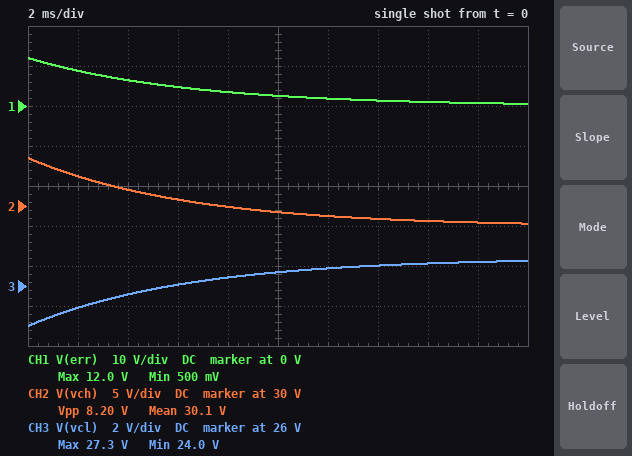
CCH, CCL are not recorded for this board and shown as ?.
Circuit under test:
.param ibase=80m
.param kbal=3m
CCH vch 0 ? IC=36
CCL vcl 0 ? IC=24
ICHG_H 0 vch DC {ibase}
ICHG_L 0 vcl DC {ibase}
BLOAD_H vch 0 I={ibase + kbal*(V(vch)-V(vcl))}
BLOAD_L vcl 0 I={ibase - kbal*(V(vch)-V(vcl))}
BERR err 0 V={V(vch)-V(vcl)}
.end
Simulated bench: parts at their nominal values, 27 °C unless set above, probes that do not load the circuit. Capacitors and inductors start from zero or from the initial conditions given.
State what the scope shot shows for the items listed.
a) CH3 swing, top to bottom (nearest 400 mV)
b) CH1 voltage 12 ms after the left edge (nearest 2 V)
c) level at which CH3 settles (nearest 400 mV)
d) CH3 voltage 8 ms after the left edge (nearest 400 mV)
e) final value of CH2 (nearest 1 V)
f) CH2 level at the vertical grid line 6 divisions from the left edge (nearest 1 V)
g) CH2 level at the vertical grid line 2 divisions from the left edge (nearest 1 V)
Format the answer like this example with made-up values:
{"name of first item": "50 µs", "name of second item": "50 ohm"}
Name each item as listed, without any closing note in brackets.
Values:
{"CH3 swing, top to bottom": "3.2 V", "CH1 voltage 12 ms after the left edge": "2 V", "level at which CH3 settles": "27.2 V", "CH3 voltage 8 ms after the left edge": "26.4 V", "final value of CH2": "28 V", "CH2 level at the vertical grid line 6 divisions from the left edge": "29 V", "CH2 level at the vertical grid line 2 divisions from the left edge": "32 V"}
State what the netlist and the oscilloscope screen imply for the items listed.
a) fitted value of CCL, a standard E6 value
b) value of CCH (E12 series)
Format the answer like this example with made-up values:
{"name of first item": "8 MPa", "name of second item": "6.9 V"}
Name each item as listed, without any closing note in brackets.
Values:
{"fitted value of CCL, a standard E6 value": "68 µF", "value of CCH": "27 µF"}
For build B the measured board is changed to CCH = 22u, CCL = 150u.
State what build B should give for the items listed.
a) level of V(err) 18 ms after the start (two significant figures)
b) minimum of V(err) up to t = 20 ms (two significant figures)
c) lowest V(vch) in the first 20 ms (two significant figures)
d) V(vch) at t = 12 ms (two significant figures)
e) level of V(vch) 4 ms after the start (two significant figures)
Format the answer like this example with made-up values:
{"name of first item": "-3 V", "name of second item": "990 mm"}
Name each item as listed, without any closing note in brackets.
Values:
{"level of V(err) 18 ms after the start": "720 mV", "minimum of V(err) up to t = 20 ms": "530 mV", "lowest V(vch) in the first 20 ms": "26 V", "V(vch) at t = 12 ms": "27 V", "level of V(vch) 4 ms after the start": "31 V"}
